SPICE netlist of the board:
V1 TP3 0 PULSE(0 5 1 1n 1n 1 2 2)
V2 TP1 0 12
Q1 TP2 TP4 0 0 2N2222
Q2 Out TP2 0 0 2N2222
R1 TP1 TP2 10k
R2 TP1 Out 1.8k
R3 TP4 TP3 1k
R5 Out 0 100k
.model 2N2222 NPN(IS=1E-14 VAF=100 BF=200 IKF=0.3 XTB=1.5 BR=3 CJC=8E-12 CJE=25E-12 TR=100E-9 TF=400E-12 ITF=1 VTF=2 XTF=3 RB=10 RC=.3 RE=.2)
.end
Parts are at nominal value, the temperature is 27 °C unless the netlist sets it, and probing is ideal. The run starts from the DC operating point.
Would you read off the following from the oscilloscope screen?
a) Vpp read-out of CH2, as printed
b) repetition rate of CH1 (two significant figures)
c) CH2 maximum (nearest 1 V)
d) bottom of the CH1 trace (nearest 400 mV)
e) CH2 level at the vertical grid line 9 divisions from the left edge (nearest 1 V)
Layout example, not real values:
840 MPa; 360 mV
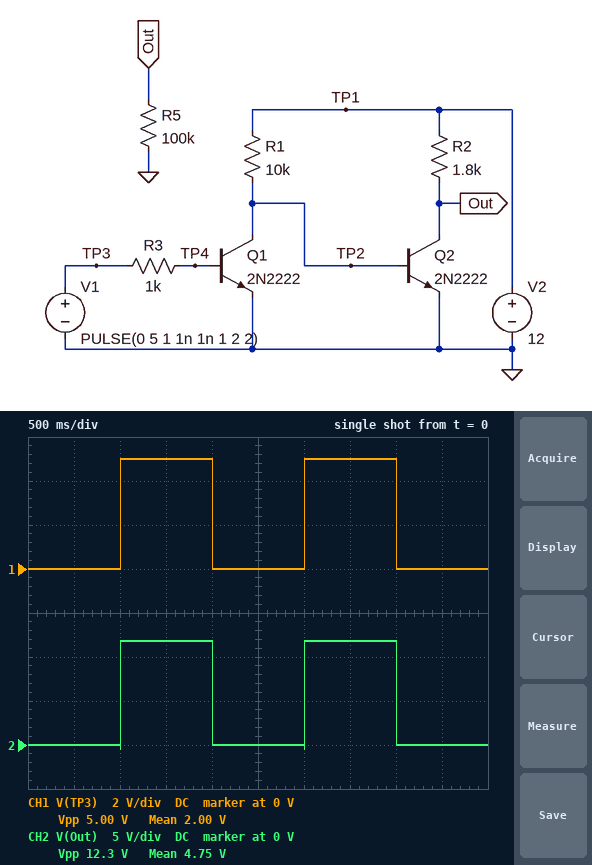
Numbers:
12.3 V; 500 mHz; 12 V; 0 V; 0 V
